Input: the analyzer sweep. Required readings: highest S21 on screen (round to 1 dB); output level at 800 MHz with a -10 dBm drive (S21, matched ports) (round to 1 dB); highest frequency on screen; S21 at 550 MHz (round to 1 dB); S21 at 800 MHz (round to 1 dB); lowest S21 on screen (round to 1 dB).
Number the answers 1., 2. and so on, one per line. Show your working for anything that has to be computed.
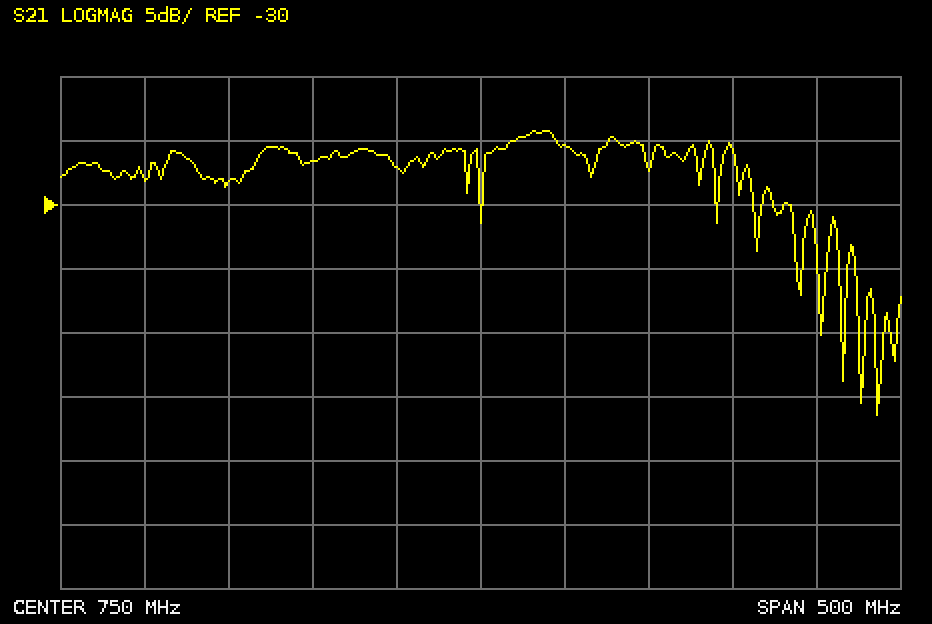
1. -24 dB
2. -10 dBm + (-25 dB) = -35 dBm
3. 1 GHz
4. -28 dB
5. -25 dB
6. -46 dB
